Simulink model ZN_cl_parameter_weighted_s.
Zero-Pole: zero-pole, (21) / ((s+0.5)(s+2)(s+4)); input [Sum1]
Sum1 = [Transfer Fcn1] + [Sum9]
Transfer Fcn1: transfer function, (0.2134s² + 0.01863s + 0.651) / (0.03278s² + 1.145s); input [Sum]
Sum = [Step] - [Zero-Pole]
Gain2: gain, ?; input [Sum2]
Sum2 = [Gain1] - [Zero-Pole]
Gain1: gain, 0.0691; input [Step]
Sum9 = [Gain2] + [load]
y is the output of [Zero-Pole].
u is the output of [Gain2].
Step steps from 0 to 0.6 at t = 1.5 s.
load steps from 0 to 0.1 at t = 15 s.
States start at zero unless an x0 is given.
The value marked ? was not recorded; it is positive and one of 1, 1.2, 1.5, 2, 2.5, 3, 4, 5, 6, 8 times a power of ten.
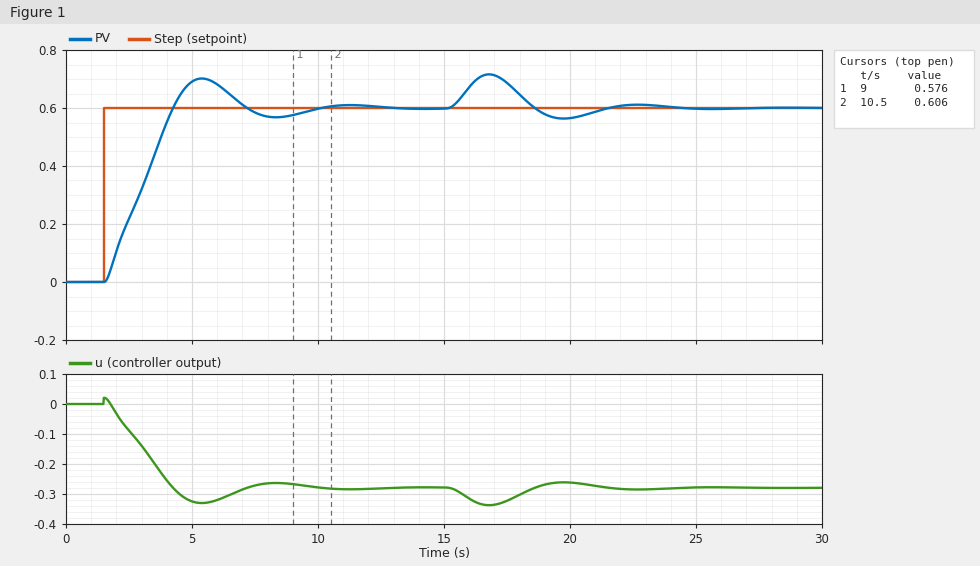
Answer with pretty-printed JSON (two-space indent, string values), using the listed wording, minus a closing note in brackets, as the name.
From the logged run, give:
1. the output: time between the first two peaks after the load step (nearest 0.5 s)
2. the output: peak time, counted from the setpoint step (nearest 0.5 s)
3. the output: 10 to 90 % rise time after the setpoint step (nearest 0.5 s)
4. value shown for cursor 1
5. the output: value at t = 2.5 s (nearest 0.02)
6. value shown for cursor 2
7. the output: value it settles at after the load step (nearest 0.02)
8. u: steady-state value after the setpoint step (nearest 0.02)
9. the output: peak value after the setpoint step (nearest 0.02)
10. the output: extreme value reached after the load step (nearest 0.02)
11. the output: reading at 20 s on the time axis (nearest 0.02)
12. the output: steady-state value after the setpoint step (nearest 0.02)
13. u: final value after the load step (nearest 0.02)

{
  "the output: time between the first two peaks after the load step": "6.0 s",
  "the output: peak time, counted from the setpoint step": "4.0 s",
  "the output: 10 to 90 % rise time after the setpoint step": "2.0 s",
  "value shown for cursor 1": "0.576",
  "the output: value at t = 2.5 s": "0.22",
  "value shown for cursor 2": "0.606",
  "the output: value it settles at after the load step": "0.60",
  "u: steady-state value after the setpoint step": "-0.28",
  "the output: peak value after the setpoint step": "0.70",
  "the output: extreme value reached after the load step": "0.72",
  "the output: reading at 20 s on the time axis": "0.56",
  "the output: steady-state value after the setpoint step": "0.60",
  "u: final value after the load step": "-0.28"
}
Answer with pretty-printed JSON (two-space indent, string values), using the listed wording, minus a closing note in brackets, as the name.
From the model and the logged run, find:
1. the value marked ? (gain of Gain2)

{
  "the value marked ?": "0.5"
}
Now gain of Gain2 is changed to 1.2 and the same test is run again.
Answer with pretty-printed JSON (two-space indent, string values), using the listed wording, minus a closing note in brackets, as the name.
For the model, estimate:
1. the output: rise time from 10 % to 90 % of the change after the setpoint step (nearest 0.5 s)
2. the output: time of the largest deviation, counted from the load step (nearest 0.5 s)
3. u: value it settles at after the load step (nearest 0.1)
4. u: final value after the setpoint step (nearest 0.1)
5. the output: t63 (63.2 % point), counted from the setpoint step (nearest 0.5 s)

{
  "the output: rise time from 10 % to 90 % of the change after the setpoint step": "4.5 s",
  "the output: time of the largest deviation, counted from the load step": "1.5 s",
  "u: value it settles at after the load step": "-0.7",
  "u: final value after the setpoint step": "-0.7",
  "the output: t63 (63.2 % point), counted from the setpoint step": "2.5 s"
}
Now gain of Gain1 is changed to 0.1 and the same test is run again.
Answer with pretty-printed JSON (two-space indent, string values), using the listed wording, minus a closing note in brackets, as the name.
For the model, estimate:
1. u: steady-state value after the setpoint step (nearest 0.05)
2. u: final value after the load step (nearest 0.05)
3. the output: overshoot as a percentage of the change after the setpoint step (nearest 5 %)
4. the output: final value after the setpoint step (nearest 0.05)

{
  "u: steady-state value after the setpoint step": "-0.25",
  "u: final value after the load step": "-0.25",
  "the output: overshoot as a percentage of the change after the setpoint step": "15 %",
  "the output: final value after the setpoint step": "0.60"
}
